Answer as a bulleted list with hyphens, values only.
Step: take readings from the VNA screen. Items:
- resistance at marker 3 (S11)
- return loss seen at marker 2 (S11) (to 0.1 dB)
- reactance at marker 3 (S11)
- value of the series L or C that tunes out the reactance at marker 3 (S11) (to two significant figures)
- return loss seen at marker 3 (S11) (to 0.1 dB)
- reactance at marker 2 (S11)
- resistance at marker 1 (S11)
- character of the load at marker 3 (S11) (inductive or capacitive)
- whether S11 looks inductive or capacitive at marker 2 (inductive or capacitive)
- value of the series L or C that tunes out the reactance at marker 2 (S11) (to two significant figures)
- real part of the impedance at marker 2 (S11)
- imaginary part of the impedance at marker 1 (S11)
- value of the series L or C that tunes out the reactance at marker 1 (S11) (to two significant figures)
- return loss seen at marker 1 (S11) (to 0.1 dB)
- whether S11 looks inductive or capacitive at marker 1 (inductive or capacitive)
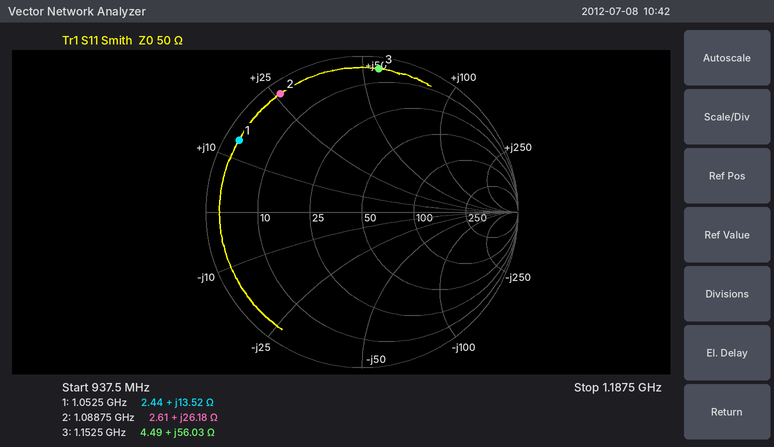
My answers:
- 4.49 Ω
- 0.7 dB
- +56.03 Ω
- 2.5 pF
- 0.7 dB
- +26.18 Ω
- 2.44 Ω
- inductive
- inductive
- 5.6 pF
- 2.61 Ω
- +13.52 Ω
- 11 pF
- 0.8 dB
- inductive
